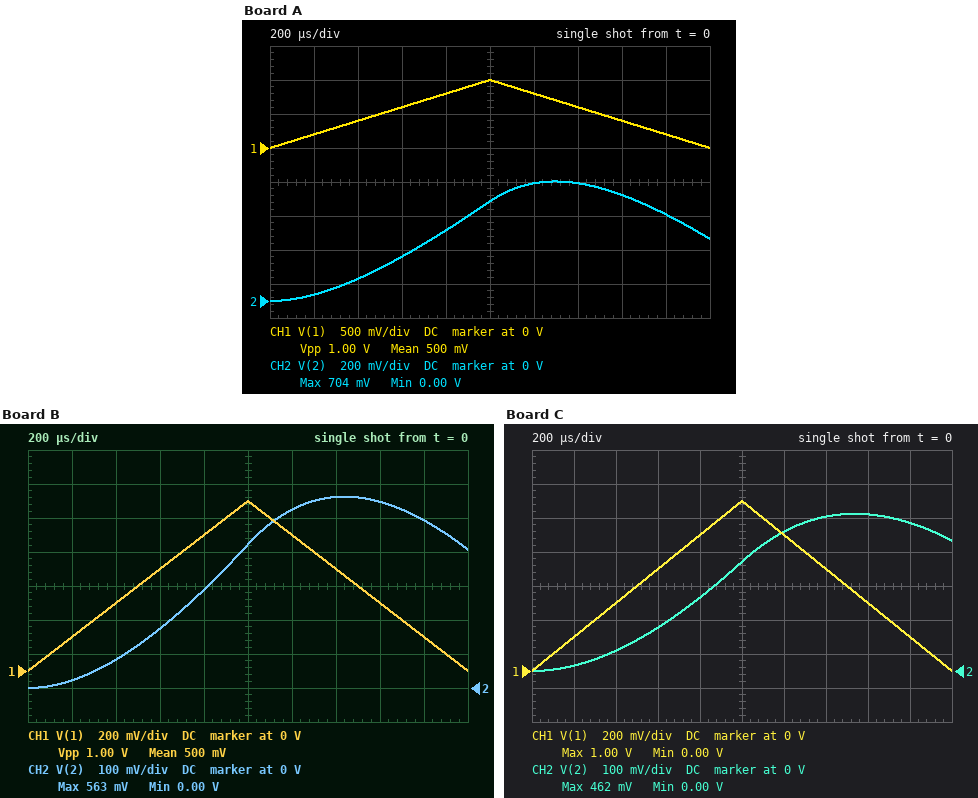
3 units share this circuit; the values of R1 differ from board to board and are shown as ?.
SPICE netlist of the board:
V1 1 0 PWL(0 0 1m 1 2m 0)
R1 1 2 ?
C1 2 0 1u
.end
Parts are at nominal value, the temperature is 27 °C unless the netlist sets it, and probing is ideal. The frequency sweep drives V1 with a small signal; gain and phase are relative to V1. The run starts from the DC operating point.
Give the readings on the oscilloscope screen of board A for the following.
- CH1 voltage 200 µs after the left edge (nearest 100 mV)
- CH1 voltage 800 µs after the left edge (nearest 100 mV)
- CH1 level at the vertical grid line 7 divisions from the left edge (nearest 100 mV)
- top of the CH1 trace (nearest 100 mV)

200 mV
800 mV
600 mV
1.0 V
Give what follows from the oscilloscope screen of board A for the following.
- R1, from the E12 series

470 Ω
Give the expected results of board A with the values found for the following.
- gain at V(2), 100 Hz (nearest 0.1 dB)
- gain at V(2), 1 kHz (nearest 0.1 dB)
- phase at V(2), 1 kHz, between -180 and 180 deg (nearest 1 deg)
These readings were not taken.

-0.4 dB
-9.9 dB
-71 deg
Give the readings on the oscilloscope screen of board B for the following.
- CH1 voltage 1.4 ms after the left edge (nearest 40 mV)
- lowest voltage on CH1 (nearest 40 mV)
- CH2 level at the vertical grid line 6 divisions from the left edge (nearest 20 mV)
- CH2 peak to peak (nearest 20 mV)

600 mV
0 V
520 mV
560 mV
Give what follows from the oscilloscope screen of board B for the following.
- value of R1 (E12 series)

820 Ω
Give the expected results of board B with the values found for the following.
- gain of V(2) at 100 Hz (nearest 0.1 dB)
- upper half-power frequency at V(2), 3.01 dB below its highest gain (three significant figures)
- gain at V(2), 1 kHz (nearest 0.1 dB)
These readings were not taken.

-1.0 dB
194 Hz
-14.4 dB
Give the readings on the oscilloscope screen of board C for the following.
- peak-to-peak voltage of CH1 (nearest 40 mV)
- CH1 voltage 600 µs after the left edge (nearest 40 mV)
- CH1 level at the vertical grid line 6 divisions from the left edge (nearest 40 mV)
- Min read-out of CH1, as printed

1.00 V
600 mV
800 mV
0.00 V
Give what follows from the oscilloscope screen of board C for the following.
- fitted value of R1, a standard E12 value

1.2 kΩ
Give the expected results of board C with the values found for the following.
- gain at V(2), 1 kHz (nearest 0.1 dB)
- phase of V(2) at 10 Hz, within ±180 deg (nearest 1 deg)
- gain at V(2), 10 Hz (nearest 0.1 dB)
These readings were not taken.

-17.6 dB
-4 deg
0 dB
